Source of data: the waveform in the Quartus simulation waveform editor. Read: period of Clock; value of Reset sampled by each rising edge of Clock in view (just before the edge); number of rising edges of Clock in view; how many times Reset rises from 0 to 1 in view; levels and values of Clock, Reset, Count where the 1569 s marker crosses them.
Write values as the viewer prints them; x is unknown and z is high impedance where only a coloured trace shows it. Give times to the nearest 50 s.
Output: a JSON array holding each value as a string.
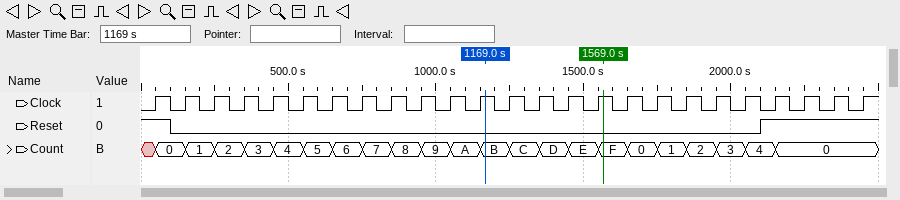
["100 s", "1 0 0 0 0 0 0 0 0 0 0 0 0 0 0 0 0 0 0 0 0 1 1 1 1", "25", "1", "Clock=1, Reset=0, Count=F"]
